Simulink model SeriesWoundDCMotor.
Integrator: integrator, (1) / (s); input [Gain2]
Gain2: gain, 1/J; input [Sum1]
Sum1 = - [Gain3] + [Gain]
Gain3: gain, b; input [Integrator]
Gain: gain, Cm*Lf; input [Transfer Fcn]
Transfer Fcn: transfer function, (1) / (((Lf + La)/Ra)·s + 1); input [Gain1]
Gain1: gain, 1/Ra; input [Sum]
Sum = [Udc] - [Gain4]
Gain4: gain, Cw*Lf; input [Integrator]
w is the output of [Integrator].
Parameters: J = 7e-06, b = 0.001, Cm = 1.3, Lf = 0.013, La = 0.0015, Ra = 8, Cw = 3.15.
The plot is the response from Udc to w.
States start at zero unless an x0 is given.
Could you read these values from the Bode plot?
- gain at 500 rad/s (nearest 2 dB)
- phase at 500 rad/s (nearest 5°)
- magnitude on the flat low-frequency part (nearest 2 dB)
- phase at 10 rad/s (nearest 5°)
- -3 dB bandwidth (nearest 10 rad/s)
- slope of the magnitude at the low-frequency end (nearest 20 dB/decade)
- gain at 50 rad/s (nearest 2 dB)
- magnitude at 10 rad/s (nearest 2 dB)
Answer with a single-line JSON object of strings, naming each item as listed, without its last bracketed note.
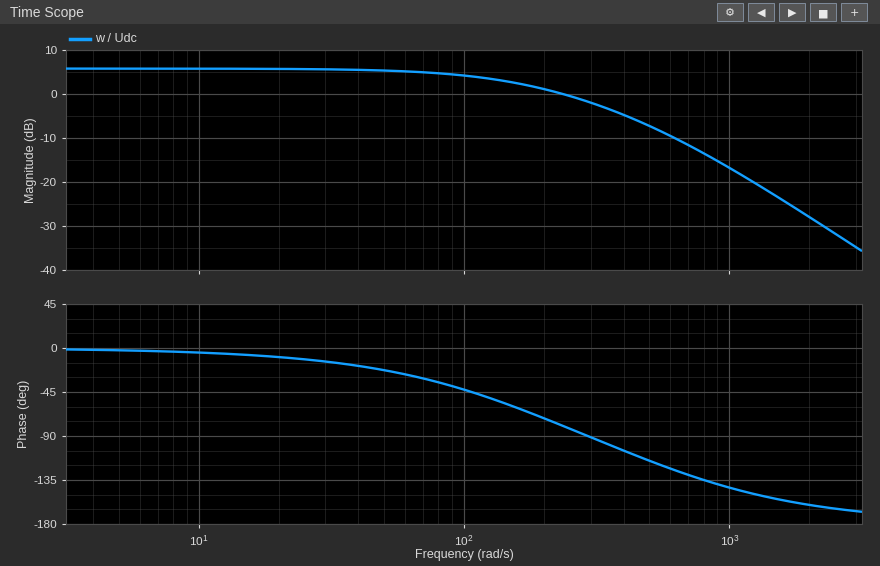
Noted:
{"gain at 500 rad/s": "-8 dB", "phase at 500 rad/s": "-115°", "magnitude on the flat low-frequency part": "6 dB", "phase at 10 rad/s": "-5°", "-3 dB bandwidth": "150 rad/s", "slope of the magnitude at the low-frequency end": "0 dB/decade", "gain at 50 rad/s": "6 dB", "magnitude at 10 rad/s": "6 dB"}
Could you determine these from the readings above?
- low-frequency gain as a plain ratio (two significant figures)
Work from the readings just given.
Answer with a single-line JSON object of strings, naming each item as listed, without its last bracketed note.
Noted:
{"low-frequency gain as a plain ratio": "2.0"}
